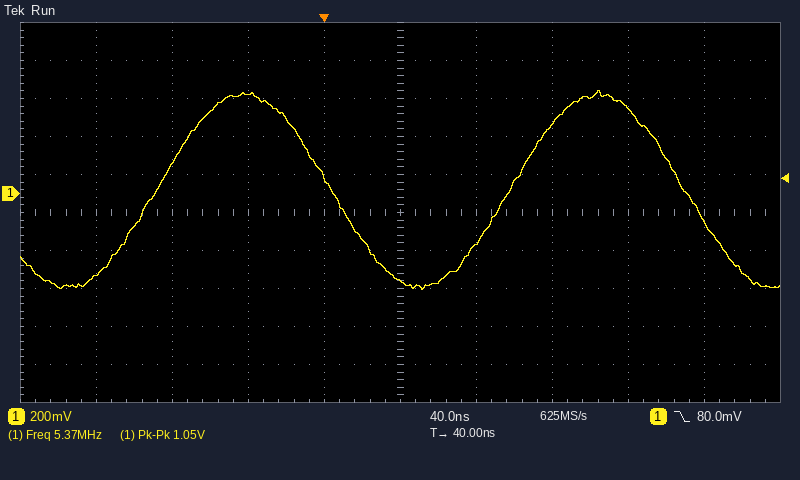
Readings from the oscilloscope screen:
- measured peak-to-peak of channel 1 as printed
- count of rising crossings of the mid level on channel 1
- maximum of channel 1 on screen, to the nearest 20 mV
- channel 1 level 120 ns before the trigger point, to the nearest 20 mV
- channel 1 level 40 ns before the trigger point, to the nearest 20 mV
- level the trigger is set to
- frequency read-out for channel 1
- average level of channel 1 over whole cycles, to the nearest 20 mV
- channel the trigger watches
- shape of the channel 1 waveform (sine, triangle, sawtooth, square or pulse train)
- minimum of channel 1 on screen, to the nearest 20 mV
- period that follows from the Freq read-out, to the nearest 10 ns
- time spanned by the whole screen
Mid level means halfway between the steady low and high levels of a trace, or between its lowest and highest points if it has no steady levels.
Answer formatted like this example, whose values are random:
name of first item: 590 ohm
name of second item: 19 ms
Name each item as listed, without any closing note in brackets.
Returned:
measured peak-to-peak of channel 1 as printed: 1.05 V
count of rising crossings of the mid level on channel 1: 2
maximum of channel 1 on screen, to the nearest 20 mV: 540 mV
channel 1 level 120 ns before the trigger point, to the nearest 20 mV: -420 mV
channel 1 level 40 ns before the trigger point, to the nearest 20 mV: 520 mV
level the trigger is set to: 80.0 mV
frequency read-out for channel 1: 5.37 MHz
average level of channel 1 over whole cycles, to the nearest 20 mV: 20 mV
channel the trigger watches: channel 1
shape of the channel 1 waveform: sine
minimum of channel 1 on screen, to the nearest 20 mV: -500 mV
period that follows from the Freq read-out, to the nearest 10 ns: 190 ns
time spanned by the whole screen: 400 ns
